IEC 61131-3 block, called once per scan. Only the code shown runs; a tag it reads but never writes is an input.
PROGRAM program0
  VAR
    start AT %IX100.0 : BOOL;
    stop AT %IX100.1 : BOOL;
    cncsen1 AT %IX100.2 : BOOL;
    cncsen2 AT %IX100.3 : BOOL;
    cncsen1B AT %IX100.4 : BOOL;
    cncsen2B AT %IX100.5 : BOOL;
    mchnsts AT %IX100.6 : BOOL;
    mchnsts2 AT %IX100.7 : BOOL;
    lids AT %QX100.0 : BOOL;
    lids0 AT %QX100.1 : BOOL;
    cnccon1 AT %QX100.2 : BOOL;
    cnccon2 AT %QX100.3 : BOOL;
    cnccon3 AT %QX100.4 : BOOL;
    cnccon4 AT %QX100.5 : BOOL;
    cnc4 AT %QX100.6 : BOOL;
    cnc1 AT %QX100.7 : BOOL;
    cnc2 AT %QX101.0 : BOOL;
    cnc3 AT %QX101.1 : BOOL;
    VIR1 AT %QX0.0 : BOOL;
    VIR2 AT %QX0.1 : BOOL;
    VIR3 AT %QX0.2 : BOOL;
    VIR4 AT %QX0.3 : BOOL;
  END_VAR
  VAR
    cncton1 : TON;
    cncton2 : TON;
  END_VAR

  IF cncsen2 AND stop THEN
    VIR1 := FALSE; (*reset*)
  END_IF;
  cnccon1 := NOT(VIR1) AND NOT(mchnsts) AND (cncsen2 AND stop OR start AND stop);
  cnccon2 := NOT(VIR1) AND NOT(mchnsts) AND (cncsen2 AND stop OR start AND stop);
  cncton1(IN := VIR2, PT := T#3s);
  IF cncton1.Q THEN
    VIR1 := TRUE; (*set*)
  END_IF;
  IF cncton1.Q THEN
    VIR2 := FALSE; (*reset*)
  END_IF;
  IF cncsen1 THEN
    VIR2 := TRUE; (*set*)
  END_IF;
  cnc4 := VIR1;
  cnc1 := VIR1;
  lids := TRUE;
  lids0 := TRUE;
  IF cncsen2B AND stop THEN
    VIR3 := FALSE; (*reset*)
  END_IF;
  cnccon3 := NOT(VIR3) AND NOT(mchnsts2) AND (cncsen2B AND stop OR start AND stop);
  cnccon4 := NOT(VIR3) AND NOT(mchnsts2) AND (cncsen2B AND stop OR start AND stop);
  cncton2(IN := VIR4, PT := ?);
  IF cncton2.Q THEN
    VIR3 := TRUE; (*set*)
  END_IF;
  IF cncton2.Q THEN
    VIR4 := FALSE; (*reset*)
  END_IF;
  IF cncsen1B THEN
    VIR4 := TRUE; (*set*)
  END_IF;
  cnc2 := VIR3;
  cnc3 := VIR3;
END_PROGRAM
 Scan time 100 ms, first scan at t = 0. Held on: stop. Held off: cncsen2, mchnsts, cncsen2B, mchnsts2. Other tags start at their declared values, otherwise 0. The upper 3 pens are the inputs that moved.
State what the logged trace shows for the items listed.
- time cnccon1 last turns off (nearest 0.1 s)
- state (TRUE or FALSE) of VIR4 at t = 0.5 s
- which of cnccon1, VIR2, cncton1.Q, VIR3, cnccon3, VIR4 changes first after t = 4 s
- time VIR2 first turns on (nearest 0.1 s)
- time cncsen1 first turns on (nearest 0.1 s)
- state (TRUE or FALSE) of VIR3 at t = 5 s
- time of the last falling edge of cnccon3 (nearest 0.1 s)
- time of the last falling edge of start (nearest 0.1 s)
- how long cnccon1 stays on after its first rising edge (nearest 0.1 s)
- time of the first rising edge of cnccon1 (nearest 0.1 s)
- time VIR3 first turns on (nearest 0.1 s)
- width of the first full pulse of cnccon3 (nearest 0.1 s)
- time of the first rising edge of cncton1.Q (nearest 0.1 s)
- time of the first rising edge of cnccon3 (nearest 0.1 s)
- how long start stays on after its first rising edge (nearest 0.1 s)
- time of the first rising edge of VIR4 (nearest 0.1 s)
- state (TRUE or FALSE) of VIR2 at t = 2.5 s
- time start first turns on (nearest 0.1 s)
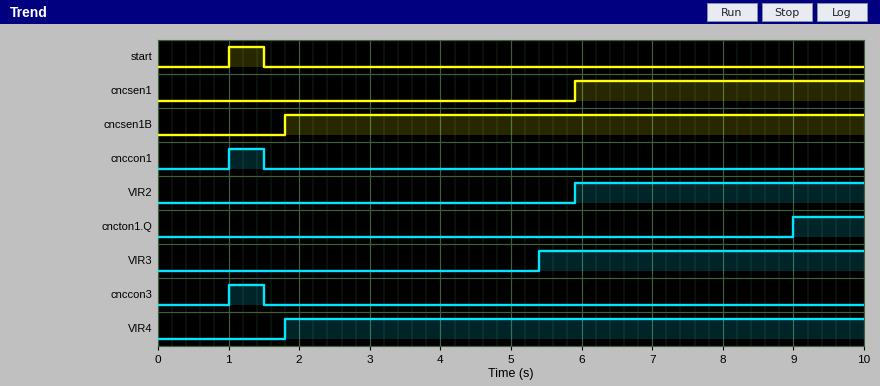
1.5 s
FALSE
VIR3
5.9 s
5.9 s
FALSE
1.5 s
1.5 s
0.5 s
1.0 s
5.4 s
0.5 s
9.0 s
1.0 s
0.5 s
1.8 s
FALSE
1.0 s
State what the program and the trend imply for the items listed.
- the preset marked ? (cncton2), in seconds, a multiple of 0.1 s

3.5 s
